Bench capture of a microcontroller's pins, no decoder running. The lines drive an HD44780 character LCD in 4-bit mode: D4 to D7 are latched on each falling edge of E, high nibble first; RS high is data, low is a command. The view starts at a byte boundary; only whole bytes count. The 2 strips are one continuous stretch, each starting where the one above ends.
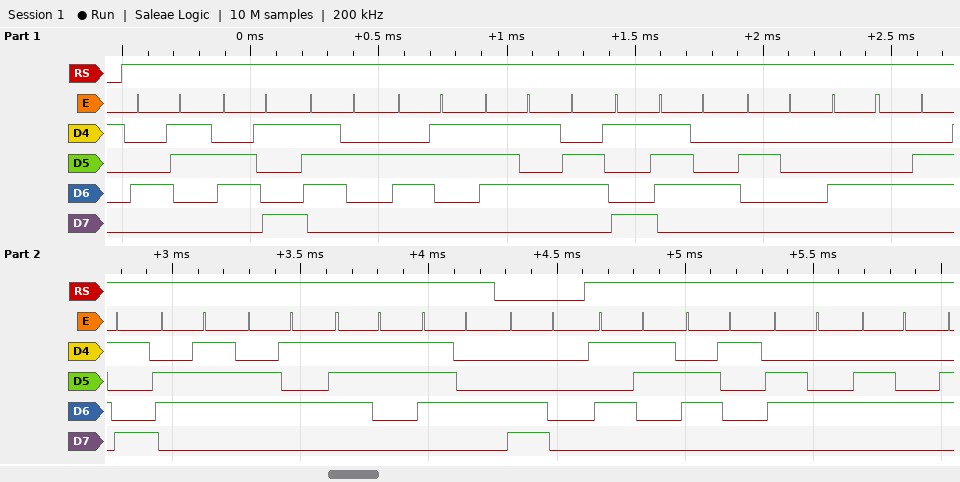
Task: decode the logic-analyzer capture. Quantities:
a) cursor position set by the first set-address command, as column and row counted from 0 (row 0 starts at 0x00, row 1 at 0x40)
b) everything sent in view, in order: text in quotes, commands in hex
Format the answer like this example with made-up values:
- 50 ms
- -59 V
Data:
- column 0, row 1
- "Circuit Digest" 0xC0 "Sadd"
